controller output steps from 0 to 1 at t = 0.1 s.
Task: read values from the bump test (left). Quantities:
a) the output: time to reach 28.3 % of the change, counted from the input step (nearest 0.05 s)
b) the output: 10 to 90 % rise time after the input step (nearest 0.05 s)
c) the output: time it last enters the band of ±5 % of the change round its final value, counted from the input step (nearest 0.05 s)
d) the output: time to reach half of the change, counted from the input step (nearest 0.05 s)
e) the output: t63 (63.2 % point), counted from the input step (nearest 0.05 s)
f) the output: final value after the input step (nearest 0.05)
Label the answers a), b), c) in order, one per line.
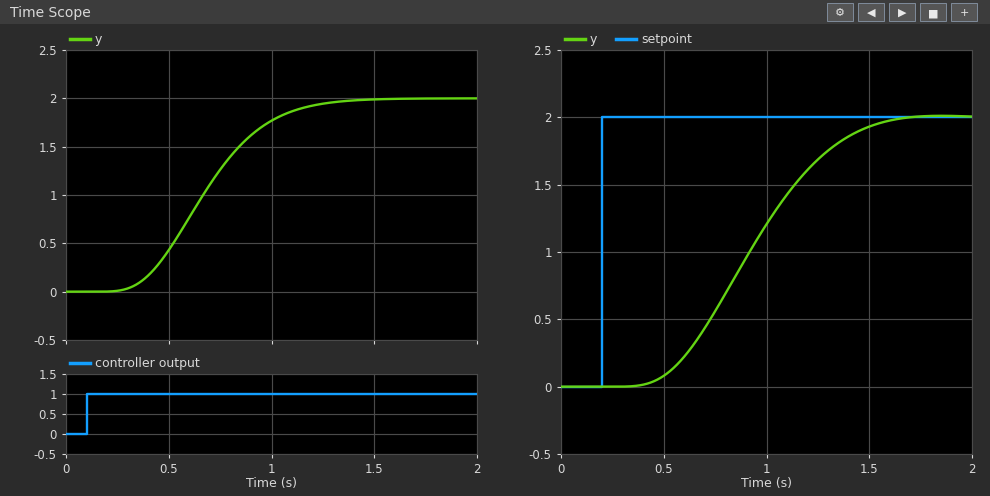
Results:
a) 0.45 s
b) 0.60 s
c) 1.05 s
d) 0.55 s
e) 0.65 s
f) 2.00
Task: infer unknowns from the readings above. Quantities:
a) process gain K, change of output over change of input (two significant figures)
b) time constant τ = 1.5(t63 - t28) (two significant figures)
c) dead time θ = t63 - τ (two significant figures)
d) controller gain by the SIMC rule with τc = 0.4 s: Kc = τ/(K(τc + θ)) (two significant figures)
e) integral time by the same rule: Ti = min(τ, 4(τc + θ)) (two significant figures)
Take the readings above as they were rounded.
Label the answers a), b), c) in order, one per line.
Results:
a) 2.0
b) 0.30 s
c) 0.35 s
d) 0.20
e) 0.30 s
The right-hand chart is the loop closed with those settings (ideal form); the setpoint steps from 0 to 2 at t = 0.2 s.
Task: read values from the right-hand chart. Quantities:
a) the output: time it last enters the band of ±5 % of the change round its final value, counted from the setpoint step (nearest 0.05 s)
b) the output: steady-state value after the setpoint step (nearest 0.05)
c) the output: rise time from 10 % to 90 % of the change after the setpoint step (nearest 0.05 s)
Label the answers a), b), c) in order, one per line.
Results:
a) 1.25 s
b) 2.00
c) 0.75 s
